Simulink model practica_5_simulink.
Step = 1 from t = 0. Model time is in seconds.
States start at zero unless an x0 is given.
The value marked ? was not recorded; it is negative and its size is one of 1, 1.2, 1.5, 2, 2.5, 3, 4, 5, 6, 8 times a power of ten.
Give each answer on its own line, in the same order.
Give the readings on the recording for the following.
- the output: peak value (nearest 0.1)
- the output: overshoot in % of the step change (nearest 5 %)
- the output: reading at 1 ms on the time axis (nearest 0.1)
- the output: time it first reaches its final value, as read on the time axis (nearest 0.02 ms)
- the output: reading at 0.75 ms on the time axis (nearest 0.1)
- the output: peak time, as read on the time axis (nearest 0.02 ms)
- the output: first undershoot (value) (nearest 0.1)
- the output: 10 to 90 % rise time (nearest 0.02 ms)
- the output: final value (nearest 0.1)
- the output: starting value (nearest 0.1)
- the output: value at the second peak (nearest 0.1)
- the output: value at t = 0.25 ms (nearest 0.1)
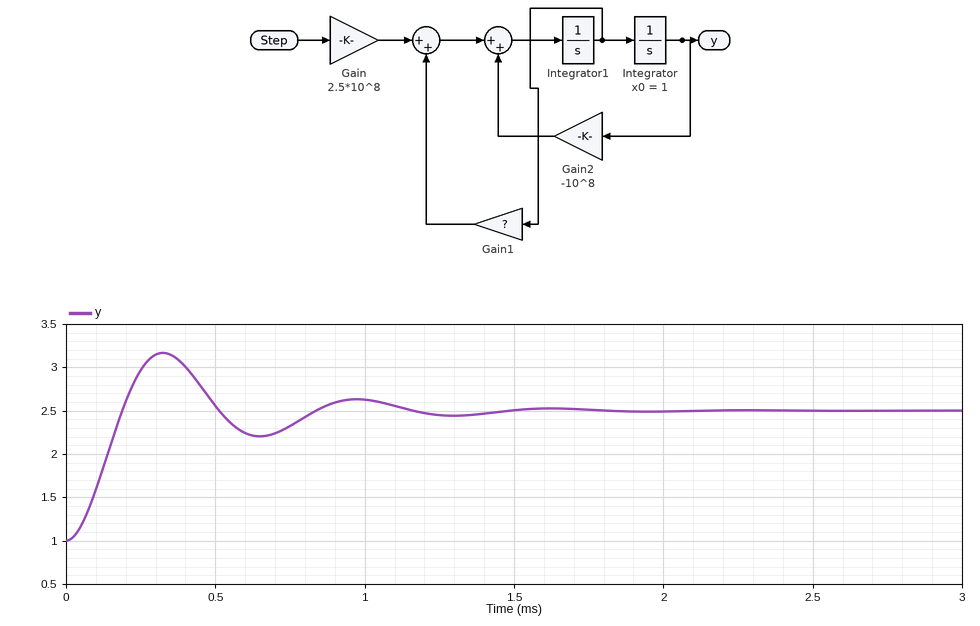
3.2
45 %
2.6
0.18 ms
2.3
0.32 ms
2.2
0.12 ms
2.5
1.0
2.6
3.0
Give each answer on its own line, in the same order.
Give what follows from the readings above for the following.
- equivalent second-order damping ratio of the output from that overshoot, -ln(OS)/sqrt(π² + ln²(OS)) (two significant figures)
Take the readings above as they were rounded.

0.25
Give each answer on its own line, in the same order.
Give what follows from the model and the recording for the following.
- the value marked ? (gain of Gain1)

-5000
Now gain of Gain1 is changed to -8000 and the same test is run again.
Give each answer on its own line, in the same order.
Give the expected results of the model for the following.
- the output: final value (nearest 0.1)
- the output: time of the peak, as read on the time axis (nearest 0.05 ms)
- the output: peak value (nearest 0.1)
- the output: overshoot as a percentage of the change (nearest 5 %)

2.5
0.35 ms
2.9
25 %
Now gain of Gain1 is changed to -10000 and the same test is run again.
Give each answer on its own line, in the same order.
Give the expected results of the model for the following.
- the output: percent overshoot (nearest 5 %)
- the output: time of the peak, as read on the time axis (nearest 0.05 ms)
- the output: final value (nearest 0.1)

15 %
0.35 ms
2.5
